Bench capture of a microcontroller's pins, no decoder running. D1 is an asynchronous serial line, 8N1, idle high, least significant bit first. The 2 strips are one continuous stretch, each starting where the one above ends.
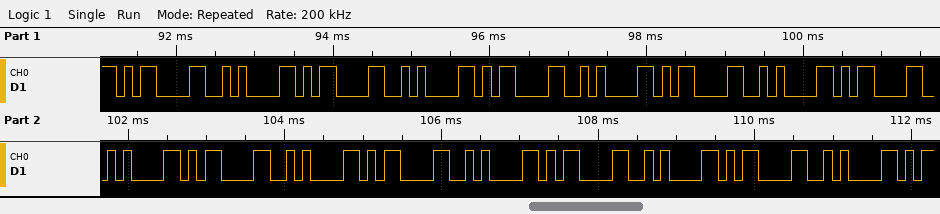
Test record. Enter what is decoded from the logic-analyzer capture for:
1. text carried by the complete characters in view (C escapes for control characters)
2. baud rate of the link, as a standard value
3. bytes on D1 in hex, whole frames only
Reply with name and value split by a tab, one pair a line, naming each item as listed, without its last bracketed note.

text carried by the complete characters in view	"\r\n\r\n\r\n\r\n\r\n\r\n\r\n\r\n\r\n"
baud rate of the link, as a standard value	9600 baud
bytes on D1 in hex, whole frames only	0x0D 0x0A 0x0D 0x0A 0x0D 0x0A 0x0D 0x0A 0x0D 0x0A 0x0D 0x0A 0x0D 0x0A 0x0D 0x0A 0x0D 0x0A
